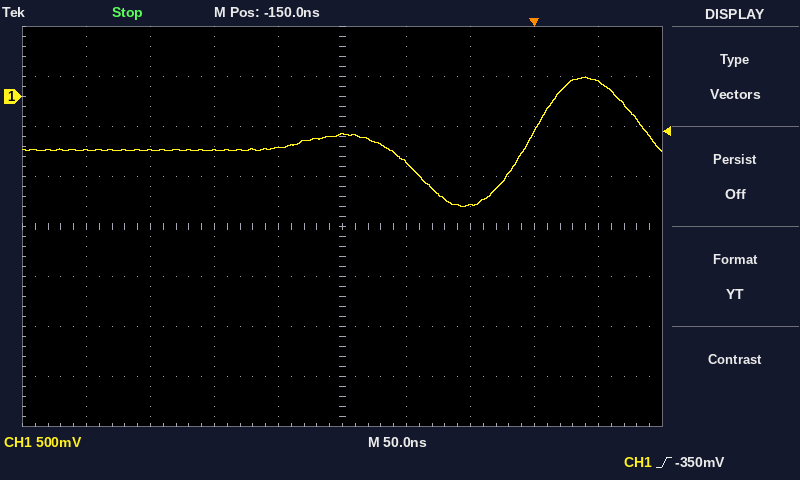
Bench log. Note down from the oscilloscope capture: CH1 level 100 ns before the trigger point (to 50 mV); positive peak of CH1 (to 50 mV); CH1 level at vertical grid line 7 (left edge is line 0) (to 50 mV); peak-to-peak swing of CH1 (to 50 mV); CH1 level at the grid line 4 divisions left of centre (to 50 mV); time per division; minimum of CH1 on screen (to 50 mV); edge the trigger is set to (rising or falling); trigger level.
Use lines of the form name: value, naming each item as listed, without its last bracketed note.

CH1 level 100 ns before the trigger point: -650 mV
positive peak of CH1: 200 mV
CH1 level at vertical grid line 7 (left edge is line 0): -1.10 V
peak-to-peak swing of CH1: 1.30 V
CH1 level at the grid line 4 divisions left of centre: -550 mV
time per division: 50 ns
minimum of CH1 on screen: -1.10 V
edge the trigger is set to: rising
trigger level: -350 mV
